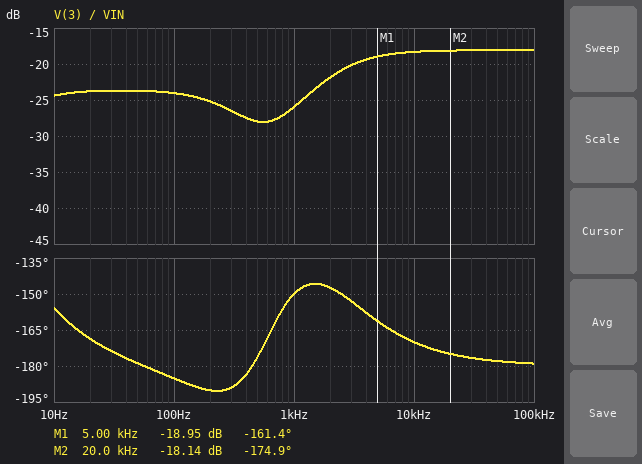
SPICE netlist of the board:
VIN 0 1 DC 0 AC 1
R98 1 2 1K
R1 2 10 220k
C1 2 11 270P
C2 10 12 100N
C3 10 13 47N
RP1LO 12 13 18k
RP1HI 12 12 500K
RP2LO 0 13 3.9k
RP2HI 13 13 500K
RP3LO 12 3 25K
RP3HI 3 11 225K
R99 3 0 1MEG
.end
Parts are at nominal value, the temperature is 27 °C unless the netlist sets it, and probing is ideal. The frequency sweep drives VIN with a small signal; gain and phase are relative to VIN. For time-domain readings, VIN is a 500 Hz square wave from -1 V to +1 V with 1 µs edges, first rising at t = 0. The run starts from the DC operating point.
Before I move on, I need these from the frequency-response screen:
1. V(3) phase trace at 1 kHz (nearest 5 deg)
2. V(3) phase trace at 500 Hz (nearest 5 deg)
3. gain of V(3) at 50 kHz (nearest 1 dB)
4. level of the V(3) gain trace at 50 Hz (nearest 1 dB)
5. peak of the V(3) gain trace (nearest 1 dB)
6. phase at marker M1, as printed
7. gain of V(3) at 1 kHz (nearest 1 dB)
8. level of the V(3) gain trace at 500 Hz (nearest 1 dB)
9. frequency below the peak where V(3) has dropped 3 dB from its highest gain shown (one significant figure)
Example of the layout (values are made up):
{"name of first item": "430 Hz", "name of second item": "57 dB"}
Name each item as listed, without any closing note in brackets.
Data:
{"V(3) phase trace at 1 kHz": "-150 deg", "V(3) phase trace at 500 Hz": "-175 deg", "gain of V(3) at 50 kHz": "-18 dB", "level of the V(3) gain trace at 50 Hz": "-24 dB", "peak of the V(3) gain trace": "-18 dB", "phase at marker M1, as printed": "-161.4 deg", "gain of V(3) at 1 kHz": "-26 dB", "level of the V(3) gain trace at 500 Hz": "-28 dB", "frequency below the peak where V(3) has dropped 3 dB from its highest gain shown": "2 kHz"}
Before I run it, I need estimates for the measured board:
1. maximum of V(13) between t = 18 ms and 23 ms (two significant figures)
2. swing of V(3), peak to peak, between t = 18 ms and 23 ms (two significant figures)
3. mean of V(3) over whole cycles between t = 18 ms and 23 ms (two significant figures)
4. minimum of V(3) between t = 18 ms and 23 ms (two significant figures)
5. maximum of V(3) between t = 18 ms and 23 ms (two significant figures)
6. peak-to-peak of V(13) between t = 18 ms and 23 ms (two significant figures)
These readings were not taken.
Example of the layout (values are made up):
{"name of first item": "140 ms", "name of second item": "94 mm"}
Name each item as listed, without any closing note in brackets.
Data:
{"maximum of V(13) between t = 18 ms and 23 ms": "38 mV", "swing of V(3), peak to peak, between t = 18 ms and 23 ms": "390 mV", "mean of V(3) over whole cycles between t = 18 ms and 23 ms": "-37 mV", "minimum of V(3) between t = 18 ms and 23 ms": "-230 mV", "maximum of V(3) between t = 18 ms and 23 ms": "160 mV", "peak-to-peak of V(13) between t = 18 ms and 23 ms": "94 mV"}
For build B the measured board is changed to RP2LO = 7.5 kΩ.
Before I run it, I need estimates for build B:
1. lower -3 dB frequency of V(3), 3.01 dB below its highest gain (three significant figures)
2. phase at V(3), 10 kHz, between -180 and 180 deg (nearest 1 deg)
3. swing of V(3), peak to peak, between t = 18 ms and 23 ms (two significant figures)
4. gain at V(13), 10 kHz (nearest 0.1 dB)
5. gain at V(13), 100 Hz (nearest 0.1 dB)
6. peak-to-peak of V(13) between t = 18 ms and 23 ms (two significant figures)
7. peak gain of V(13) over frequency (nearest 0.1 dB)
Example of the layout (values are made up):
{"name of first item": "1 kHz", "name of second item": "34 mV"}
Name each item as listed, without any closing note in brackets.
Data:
{"lower -3 dB frequency of V(3), 3.01 dB below its highest gain": "2.23 kHz", "phase at V(3), 10 kHz, between -180 and 180 deg": "-171 deg", "swing of V(3), peak to peak, between t = 18 ms and 23 ms": "460 mV", "gain at V(13), 10 kHz": "-24.8 dB", "gain at V(13), 100 Hz": "-30.1 dB", "peak-to-peak of V(13) between t = 18 ms and 23 ms": "170 mV", "peak gain of V(13) over frequency": "-24.6 dB"}
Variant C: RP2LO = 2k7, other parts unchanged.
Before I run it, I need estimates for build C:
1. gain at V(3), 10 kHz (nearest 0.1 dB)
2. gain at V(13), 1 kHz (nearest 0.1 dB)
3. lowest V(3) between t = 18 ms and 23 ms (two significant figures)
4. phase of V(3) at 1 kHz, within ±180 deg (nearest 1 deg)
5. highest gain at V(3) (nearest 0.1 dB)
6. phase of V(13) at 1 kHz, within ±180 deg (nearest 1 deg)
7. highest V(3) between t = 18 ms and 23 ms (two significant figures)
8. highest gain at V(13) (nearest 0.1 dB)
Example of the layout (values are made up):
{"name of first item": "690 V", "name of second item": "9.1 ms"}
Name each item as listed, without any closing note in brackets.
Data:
{"gain at V(3), 10 kHz": "-18.9 dB", "gain at V(13), 1 kHz": "-37.1 dB", "lowest V(3) between t = 18 ms and 23 ms": "-220 mV", "phase of V(3) at 1 kHz, within ±180 deg": "-148 deg", "highest gain at V(3)": "-18.7 dB", "phase of V(13) at 1 kHz, within ±180 deg": "-164 deg", "highest V(3) between t = 18 ms and 23 ms": "150 mV", "highest gain at V(13)": "-33.1 dB"}
